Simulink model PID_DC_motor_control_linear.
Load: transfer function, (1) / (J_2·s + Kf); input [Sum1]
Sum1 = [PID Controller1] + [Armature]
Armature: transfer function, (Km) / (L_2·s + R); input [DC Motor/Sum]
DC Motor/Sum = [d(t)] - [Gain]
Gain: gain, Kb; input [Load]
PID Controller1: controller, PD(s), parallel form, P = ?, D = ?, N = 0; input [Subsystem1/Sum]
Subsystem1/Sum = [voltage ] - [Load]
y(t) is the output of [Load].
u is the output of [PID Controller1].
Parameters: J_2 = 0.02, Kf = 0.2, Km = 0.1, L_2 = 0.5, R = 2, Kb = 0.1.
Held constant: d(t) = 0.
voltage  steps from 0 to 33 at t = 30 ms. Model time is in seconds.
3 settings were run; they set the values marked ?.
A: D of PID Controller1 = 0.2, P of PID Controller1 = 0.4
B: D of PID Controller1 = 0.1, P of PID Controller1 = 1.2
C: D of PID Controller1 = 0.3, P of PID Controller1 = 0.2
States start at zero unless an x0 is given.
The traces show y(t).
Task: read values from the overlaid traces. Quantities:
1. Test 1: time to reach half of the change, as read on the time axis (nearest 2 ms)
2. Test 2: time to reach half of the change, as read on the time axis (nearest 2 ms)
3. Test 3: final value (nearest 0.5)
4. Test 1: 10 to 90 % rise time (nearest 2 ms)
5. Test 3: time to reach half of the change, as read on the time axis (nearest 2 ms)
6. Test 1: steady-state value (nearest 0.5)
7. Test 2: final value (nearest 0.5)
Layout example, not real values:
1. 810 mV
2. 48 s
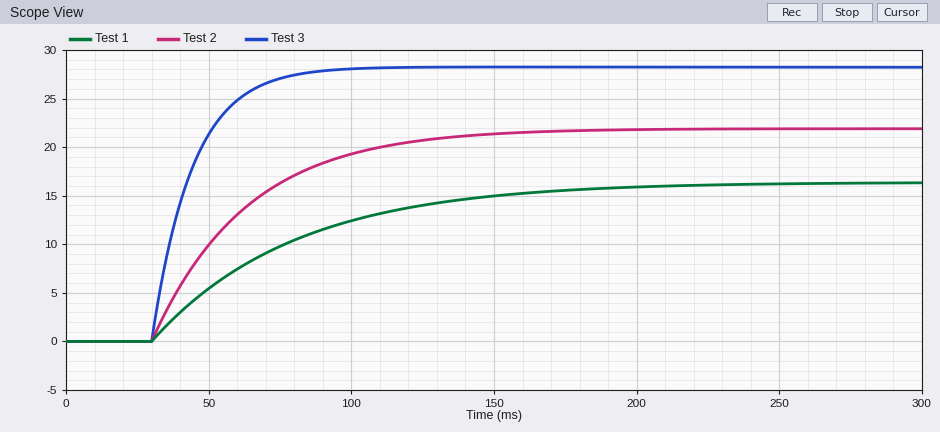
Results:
1. 64 ms
2. 52 ms
3. 28.0
4. 106 ms
5. 40 ms
6. 16.5
7. 22.0
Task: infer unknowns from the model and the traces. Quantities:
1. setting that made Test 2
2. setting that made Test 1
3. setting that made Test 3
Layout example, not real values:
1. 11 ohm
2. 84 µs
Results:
1. A
2. C
3. B
